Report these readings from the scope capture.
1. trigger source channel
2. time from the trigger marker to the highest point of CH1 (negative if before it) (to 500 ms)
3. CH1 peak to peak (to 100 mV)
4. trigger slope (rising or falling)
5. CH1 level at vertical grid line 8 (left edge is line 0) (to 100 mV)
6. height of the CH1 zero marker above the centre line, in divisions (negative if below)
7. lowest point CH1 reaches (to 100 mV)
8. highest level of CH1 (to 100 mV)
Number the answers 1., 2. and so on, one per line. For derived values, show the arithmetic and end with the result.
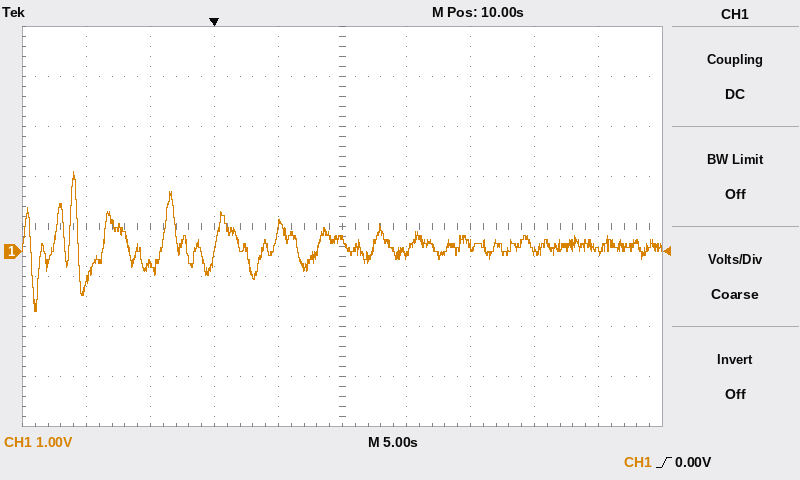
1. CH1
2. -11.0 s
3. 1.6 V − (-1.2 V) = 2.8 V
4. rising
5. 0.0 V
6. -0.5 div
7. -1.2 V
8. 1.6 V
